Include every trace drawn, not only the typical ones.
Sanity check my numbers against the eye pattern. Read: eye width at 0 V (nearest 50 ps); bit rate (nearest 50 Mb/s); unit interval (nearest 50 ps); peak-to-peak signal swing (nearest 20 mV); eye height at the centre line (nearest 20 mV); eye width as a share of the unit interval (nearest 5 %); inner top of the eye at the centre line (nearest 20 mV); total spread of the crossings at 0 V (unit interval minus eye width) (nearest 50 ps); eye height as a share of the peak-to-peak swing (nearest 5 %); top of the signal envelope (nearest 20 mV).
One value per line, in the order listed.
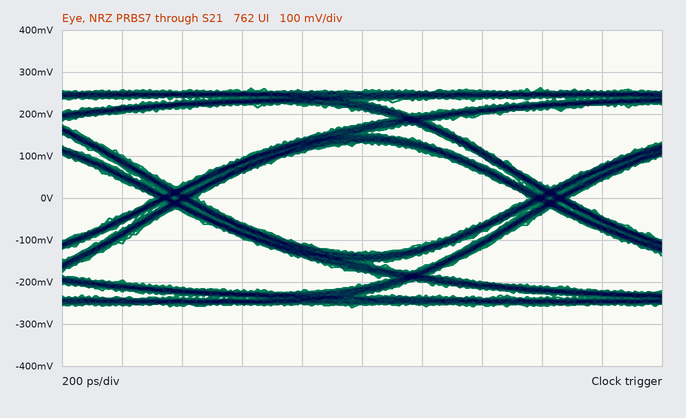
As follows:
1.10 ns
800 Mb/s
1.25 ns
520 mV
260 mV
90 %
140 mV
150 ps
50 %
260 mV
